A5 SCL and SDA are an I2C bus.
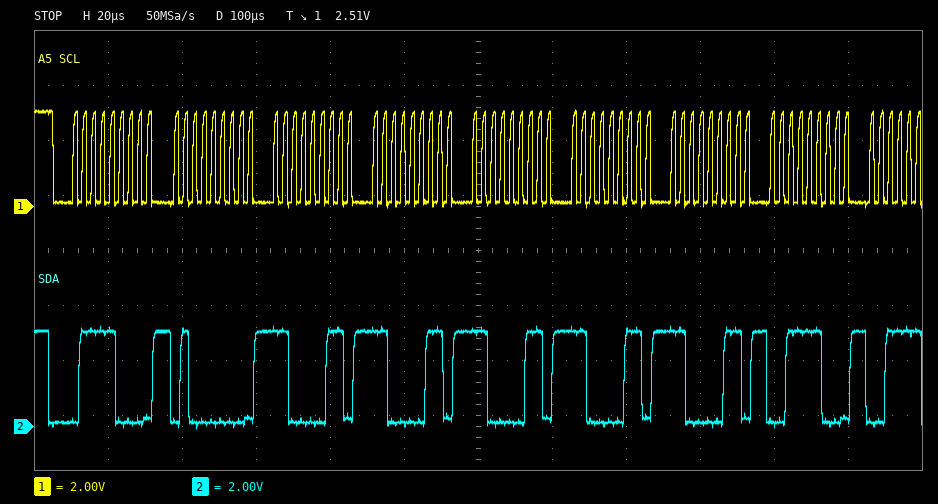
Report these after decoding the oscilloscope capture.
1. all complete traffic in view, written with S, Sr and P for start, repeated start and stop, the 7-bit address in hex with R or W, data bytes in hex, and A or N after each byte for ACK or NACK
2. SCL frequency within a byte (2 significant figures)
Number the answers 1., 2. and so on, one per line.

1. S 3CW A 40 A C3 A C3 A C3 A C3 A C3 A 3C A
2. 400 kHz
